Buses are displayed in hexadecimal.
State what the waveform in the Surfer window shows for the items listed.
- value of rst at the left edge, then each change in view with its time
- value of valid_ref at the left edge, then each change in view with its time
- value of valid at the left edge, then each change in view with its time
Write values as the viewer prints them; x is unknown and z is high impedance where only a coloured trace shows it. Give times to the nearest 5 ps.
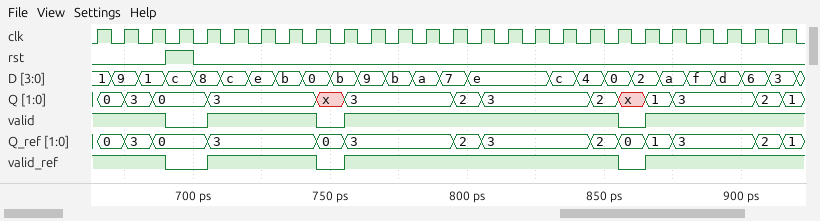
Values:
0, 1 at 690 ps, 0 at 700 ps
1, 0 at 690 ps, 1 at 705 ps, 0 at 745 ps, 1 at 755 ps, 0 at 855 ps, 1 at 865 ps
1, 0 at 690 ps, 1 at 705 ps, 0 at 745 ps, 1 at 755 ps, 0 at 855 ps, 1 at 865 ps
